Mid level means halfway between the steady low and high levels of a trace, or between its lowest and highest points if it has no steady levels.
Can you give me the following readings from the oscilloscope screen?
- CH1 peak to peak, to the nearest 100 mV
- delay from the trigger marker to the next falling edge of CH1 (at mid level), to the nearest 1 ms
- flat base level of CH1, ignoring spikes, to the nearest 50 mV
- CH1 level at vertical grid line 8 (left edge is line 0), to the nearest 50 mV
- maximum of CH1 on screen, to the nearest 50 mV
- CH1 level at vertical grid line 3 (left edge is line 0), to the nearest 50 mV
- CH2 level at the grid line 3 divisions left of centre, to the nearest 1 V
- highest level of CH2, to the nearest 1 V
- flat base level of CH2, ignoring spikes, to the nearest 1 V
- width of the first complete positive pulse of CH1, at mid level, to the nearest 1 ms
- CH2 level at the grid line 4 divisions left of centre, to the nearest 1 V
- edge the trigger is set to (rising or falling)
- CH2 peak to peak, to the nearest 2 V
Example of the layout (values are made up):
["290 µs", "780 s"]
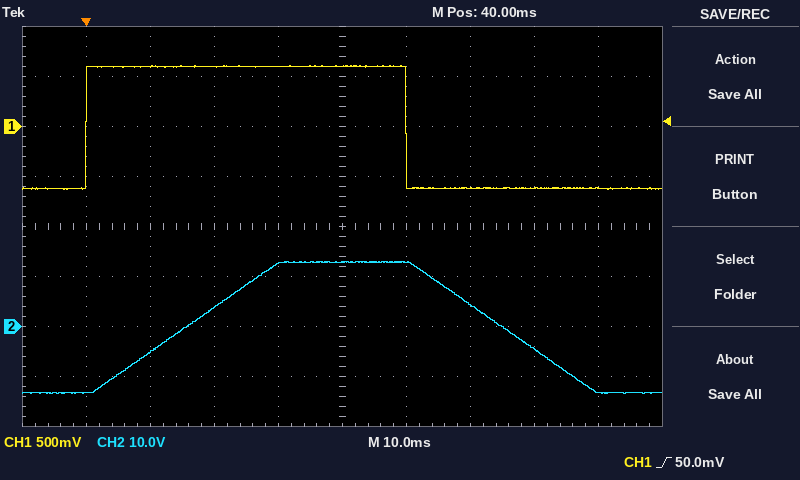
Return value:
["1.20 V", "50 ms", "-600 mV", "-600 mV", "600 mV", "600 mV", "-5 V", "13 V", "-13 V", "50 ms", "-13 V", "rising", "26 V"]
